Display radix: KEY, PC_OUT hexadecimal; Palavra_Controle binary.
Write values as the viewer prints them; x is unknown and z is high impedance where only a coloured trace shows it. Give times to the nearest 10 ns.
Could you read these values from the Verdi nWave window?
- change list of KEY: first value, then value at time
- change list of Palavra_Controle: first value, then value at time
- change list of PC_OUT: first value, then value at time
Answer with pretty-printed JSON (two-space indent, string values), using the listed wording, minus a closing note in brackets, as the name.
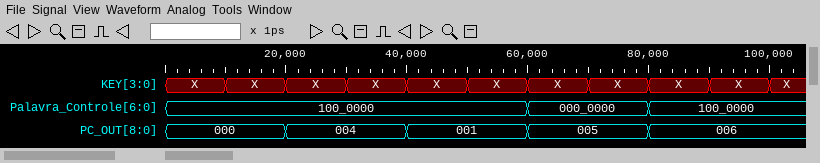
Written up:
{
  "change list of KEY: first value, then value at time": "X, X at 10 ns, X at 20 ns, X at 30 ns, X at 40 ns, X at 50 ns, X at 60 ns, X at 70 ns, X at 80 ns, X at 90 ns, X at 100 ns",
  "change list of Palavra_Controle: first value, then value at time": "100_0000, 000_0000 at 60 ns, 100_0000 at 80 ns",
  "change list of PC_OUT: first value, then value at time": "000, 004 at 20 ns, 001 at 40 ns, 005 at 60 ns, 006 at 80 ns"
}
